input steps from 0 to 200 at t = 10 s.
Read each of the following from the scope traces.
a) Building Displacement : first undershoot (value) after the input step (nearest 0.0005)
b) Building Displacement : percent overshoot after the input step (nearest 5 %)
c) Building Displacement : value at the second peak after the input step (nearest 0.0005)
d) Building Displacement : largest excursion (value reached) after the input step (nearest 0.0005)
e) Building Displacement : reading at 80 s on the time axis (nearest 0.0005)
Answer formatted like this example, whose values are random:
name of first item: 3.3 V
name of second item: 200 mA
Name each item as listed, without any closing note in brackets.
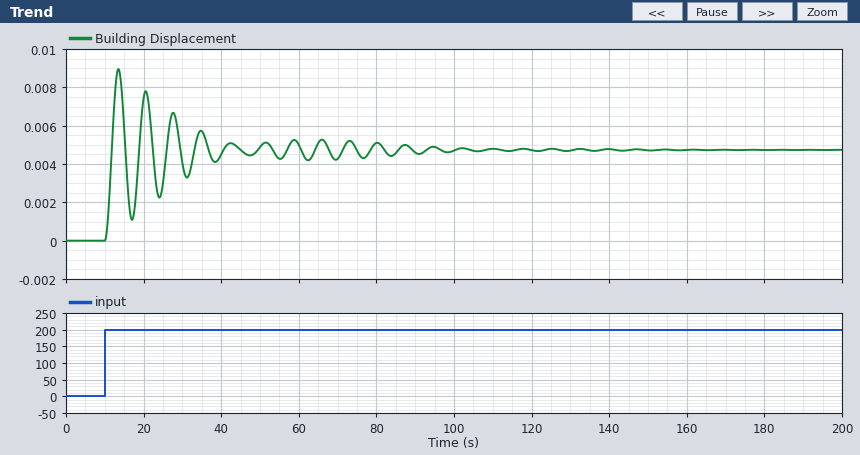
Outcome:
Building Displacement : first undershoot (value) after the input step: 0.0010
Building Displacement : percent overshoot after the input step: 90 %
Building Displacement : value at the second peak after the input step: 0.0080
Building Displacement : largest excursion (value reached) after the input step: 0.0090
Building Displacement : reading at 80 s on the time axis: 0.0050
